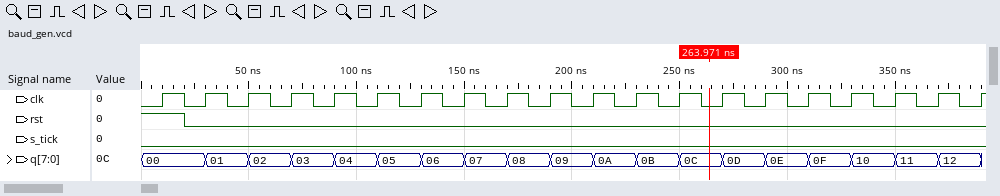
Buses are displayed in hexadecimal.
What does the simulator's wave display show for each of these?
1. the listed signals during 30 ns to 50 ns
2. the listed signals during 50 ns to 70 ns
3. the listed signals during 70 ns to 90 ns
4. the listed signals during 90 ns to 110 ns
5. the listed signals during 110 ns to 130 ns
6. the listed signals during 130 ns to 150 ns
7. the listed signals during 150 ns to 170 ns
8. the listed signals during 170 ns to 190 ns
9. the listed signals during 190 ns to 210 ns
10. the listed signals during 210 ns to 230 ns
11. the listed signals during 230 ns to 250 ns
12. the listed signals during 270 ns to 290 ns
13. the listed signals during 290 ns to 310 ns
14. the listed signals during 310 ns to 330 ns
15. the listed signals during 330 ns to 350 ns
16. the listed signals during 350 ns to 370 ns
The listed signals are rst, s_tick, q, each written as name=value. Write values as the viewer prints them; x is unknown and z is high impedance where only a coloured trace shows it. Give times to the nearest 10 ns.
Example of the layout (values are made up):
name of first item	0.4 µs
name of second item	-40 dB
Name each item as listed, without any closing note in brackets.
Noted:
the listed signals during 30 ns to 50 ns	rst=0, s_tick=0, q=01
the listed signals during 50 ns to 70 ns	rst=0, s_tick=0, q=02
the listed signals during 70 ns to 90 ns	rst=0, s_tick=0, q=03
the listed signals during 90 ns to 110 ns	rst=0, s_tick=0, q=04
the listed signals during 110 ns to 130 ns	rst=0, s_tick=0, q=05
the listed signals during 130 ns to 150 ns	rst=0, s_tick=0, q=06
the listed signals during 150 ns to 170 ns	rst=0, s_tick=0, q=07
the listed signals during 170 ns to 190 ns	rst=0, s_tick=0, q=08
the listed signals during 190 ns to 210 ns	rst=0, s_tick=0, q=09
the listed signals during 210 ns to 230 ns	rst=0, s_tick=0, q=0A
the listed signals during 230 ns to 250 ns	rst=0, s_tick=0, q=0B
the listed signals during 270 ns to 290 ns	rst=0, s_tick=0, q=0D
the listed signals during 290 ns to 310 ns	rst=0, s_tick=0, q=0E
the listed signals during 310 ns to 330 ns	rst=0, s_tick=0, q=0F
the listed signals during 330 ns to 350 ns	rst=0, s_tick=0, q=10
the listed signals during 350 ns to 370 ns	rst=0, s_tick=0, q=11
